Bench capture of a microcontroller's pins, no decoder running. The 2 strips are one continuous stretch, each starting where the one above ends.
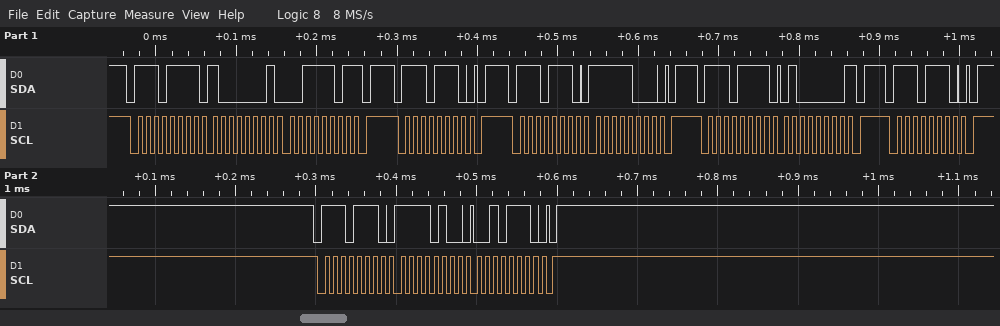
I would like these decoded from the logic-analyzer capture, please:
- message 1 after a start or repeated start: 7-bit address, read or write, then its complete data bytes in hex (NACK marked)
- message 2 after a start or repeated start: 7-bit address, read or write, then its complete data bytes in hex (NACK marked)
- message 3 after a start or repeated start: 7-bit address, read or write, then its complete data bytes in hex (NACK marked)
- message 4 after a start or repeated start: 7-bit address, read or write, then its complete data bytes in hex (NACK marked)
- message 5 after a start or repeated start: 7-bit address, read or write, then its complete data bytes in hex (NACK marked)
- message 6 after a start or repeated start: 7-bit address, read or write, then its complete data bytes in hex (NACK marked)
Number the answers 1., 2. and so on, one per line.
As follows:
1. 0x77 read: 81 3D NACK
2. 0x77 write
3. 0x77 write: F8
4. 0x77 read: 40 NACK
5. 0x77 write
6. 0x77 write: F4 2E
